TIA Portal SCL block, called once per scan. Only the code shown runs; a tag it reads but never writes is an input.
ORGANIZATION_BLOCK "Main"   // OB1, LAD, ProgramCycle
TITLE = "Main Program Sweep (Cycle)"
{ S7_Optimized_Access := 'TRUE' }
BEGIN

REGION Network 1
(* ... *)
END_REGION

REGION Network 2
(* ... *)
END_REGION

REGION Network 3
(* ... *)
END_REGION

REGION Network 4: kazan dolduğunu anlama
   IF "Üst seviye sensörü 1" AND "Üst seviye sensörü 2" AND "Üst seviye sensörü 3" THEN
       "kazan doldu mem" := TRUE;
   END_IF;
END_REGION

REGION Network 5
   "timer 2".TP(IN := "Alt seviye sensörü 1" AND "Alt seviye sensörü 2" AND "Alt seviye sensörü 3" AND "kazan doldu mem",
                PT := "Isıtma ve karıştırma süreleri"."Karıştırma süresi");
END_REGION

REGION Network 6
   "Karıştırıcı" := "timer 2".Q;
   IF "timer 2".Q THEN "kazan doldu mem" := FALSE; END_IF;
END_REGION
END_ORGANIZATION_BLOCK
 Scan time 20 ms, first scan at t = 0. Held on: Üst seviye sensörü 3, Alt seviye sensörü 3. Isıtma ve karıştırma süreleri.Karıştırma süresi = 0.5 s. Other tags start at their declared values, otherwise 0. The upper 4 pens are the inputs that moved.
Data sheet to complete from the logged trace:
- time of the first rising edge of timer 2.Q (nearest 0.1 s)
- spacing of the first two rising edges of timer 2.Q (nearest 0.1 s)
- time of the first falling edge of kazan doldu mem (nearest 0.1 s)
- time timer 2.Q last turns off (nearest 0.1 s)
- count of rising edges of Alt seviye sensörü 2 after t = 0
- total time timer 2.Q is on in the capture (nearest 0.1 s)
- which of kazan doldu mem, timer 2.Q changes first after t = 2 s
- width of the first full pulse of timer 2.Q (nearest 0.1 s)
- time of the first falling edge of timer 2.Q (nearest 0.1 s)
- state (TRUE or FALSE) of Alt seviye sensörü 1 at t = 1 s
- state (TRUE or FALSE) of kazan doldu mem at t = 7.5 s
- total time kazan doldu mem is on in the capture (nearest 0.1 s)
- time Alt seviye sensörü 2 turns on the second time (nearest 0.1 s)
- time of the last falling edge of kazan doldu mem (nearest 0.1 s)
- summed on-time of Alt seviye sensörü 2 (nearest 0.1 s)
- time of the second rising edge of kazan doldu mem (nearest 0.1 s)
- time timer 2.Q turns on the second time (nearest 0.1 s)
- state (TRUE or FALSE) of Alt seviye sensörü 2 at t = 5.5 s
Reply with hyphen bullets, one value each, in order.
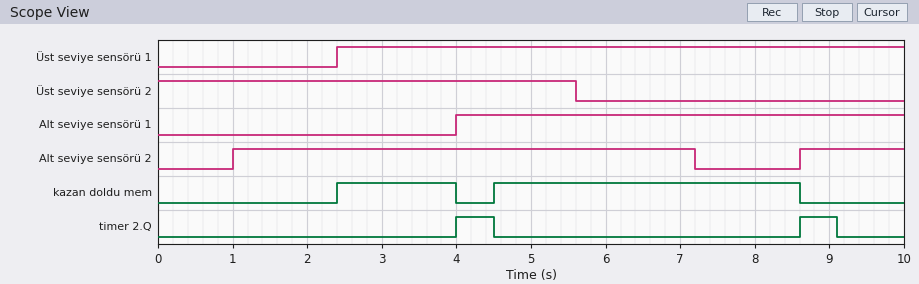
- 4.0 s
- 4.6 s
- 4.0 s
- 9.1 s
- 2
- 1.0 s
- kazan doldu mem
- 0.5 s
- 4.5 s
- FALSE
- TRUE
- 5.7 s
- 8.6 s
- 8.6 s
- 7.6 s
- 4.5 s
- 8.6 s
- TRUE
